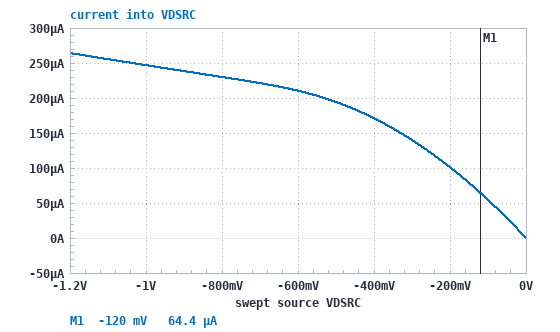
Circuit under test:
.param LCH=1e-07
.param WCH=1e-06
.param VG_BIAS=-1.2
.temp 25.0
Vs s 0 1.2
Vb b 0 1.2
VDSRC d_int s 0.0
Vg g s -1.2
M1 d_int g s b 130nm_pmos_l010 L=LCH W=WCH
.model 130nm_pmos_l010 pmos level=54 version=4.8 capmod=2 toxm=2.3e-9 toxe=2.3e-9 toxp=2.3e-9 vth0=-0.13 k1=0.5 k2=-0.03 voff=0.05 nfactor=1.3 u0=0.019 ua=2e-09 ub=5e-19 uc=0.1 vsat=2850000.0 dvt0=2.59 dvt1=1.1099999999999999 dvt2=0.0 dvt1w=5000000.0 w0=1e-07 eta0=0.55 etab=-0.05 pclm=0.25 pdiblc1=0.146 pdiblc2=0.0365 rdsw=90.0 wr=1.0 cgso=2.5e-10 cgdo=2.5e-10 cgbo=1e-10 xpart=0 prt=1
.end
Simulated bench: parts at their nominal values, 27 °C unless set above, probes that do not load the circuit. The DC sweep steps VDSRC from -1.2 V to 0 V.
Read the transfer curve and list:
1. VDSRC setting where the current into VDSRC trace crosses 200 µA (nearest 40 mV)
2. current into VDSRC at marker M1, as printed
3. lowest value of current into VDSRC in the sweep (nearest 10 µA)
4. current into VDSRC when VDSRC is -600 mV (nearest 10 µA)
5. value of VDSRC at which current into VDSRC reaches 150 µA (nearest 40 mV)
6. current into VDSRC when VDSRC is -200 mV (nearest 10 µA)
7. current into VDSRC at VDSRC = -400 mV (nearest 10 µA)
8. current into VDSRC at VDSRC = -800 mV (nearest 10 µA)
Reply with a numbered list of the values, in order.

1. -520 mV
2. 64.4 µA
3. 0 A
4. 210 µA
5. -320 mV
6. 100 µA
7. 170 µA
8. 230 µA
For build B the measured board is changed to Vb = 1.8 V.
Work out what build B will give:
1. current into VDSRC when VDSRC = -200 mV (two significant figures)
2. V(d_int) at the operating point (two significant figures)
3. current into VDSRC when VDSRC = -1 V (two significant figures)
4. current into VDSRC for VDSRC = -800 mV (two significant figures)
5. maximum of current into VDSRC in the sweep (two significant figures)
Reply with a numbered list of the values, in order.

1. 1.3 mA
2. 1.2 V
3. 3.3 mA
4. 3.0 mA
5. 3.6 mA
